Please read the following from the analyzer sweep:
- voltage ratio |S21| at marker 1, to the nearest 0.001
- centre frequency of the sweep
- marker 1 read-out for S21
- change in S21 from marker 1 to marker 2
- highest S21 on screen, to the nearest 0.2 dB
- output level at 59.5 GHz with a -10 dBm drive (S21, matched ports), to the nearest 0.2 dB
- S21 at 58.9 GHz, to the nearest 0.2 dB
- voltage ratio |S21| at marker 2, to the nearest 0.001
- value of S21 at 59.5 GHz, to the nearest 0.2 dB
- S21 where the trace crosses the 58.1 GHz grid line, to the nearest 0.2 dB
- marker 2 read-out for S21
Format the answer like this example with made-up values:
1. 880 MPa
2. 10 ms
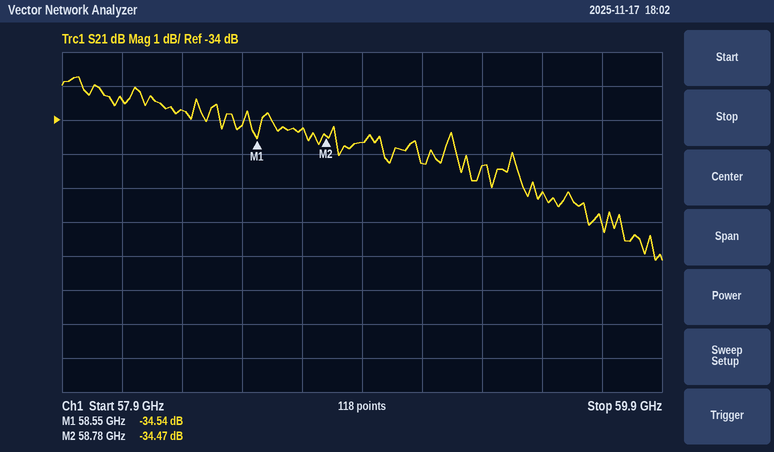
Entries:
1. 0.019
2. 58.9 GHz
3. -34.54 dB
4. 0.07 dB
5. -32.8 dB
6. -46.2 dBm
7. -34.6 dB
8. 0.019
9. -36.2 dB
10. -33.4 dB
11. -34.47 dB
